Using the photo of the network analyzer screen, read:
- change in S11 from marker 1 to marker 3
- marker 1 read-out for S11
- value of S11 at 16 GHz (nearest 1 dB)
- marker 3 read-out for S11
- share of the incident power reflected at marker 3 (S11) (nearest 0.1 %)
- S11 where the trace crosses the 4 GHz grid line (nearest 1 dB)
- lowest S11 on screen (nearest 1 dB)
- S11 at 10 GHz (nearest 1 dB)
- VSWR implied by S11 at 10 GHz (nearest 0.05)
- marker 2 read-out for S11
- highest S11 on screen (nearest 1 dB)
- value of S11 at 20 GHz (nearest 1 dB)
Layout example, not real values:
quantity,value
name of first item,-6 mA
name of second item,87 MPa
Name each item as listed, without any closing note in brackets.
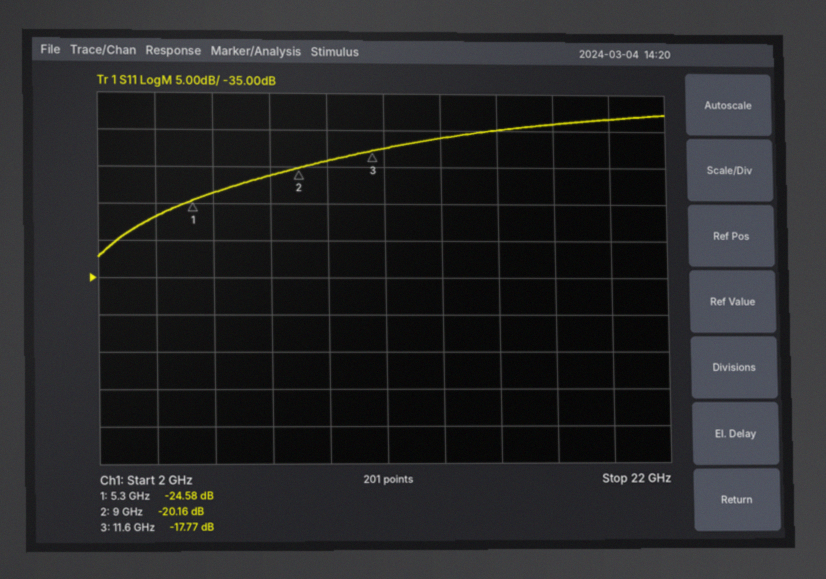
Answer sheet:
quantity,value
change in S11 from marker 1 to marker 3,6.81 dB
marker 1 read-out for S11,-24.58 dB
value of S11 at 16 GHz,-15 dB
marker 3 read-out for S11,-17.77 dB
share of the incident power reflected at marker 3 (S11),1.7 %
S11 where the trace crosses the 4 GHz grid line,-27 dB
lowest S11 on screen,-32 dB
S11 at 10 GHz,-19 dB
VSWR implied by S11 at 10 GHz,1.25
marker 2 read-out for S11,-20.16 dB
highest S11 on screen,-13 dB
value of S11 at 20 GHz,-13 dB
